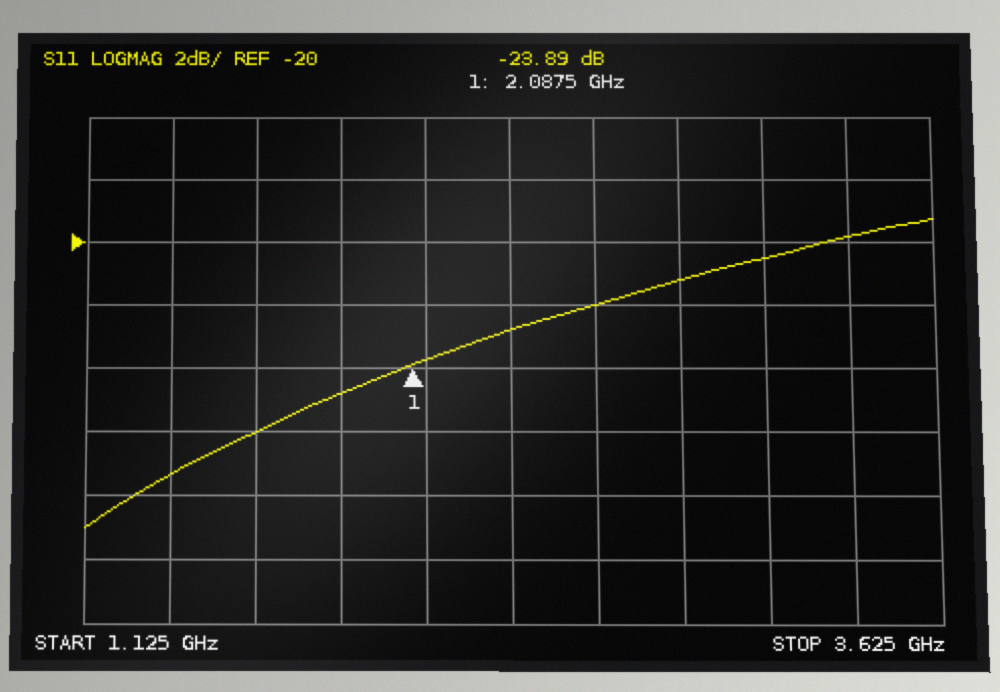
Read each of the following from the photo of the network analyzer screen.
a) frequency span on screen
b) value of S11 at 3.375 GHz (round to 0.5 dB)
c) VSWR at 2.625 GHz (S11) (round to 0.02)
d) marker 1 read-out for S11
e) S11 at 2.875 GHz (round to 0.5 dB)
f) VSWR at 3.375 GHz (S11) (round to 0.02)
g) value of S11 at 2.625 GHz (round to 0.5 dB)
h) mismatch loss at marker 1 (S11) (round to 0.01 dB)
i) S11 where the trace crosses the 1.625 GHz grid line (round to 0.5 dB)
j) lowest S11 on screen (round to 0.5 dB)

2.5 GHz
-20.0 dB
1.18
-23.89 dB
-21.0 dB
1.22
-22.0 dB
0.02 dB
-26.0 dB
-29.0 dB
